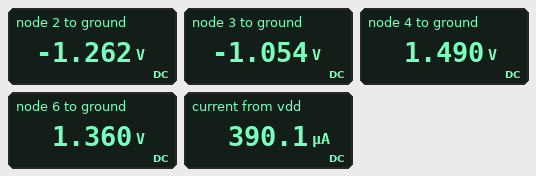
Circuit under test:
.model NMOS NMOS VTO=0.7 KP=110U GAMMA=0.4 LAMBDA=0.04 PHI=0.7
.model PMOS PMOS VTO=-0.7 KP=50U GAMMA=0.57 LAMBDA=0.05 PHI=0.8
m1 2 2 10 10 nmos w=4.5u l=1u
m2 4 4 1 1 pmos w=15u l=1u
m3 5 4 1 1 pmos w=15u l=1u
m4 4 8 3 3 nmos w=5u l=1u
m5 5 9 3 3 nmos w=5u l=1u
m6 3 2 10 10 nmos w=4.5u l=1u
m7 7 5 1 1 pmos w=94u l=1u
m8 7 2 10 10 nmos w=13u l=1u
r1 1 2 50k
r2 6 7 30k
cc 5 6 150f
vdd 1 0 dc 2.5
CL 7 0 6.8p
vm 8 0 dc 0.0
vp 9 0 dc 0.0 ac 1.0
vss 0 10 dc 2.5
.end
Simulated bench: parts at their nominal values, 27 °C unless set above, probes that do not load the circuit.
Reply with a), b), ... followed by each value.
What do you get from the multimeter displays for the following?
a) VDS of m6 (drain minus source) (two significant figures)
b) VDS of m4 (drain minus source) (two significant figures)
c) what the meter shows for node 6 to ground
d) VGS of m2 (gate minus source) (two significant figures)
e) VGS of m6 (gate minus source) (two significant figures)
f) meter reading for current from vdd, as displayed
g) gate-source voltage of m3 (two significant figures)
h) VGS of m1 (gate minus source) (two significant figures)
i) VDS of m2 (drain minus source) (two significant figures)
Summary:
a) 1.4 V
b) 2.5 V
c) 1.360 V
d) -1.0 V
e) 1.2 V
f) 390.1 µA
g) -1.0 V
h) 1.2 V
i) -1.0 V
